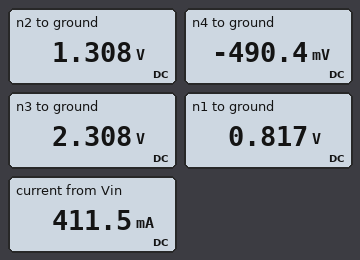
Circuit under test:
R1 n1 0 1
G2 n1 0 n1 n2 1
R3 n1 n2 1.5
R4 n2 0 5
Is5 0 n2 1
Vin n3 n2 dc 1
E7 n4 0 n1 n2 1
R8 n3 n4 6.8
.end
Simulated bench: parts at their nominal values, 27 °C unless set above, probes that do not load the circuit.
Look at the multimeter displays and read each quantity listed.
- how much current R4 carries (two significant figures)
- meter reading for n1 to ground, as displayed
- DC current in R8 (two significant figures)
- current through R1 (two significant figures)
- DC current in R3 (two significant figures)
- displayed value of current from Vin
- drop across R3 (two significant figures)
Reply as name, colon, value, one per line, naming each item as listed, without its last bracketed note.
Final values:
how much current R4 carries: 260 mA
meter reading for n1 to ground, as displayed: 0.817 V
DC current in R8: 410 mA
current through R1: 820 mA
DC current in R3: 330 mA
displayed value of current from Vin: 411.5 mA
drop across R3: 490 mV
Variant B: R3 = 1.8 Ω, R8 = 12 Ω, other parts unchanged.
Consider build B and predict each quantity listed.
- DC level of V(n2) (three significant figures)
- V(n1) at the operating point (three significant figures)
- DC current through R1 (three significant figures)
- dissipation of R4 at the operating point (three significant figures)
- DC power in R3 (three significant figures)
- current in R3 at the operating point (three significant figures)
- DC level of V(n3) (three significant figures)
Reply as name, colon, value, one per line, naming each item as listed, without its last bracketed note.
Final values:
DC level of V(n2): 1.72 V
V(n1) at the operating point: 1.05 V
DC current through R1: 1.05 A
dissipation of R4 at the operating point: 591 mW
DC power in R3: 251 mW
current in R3 at the operating point: 374 mA
DC level of V(n3): 2.72 V
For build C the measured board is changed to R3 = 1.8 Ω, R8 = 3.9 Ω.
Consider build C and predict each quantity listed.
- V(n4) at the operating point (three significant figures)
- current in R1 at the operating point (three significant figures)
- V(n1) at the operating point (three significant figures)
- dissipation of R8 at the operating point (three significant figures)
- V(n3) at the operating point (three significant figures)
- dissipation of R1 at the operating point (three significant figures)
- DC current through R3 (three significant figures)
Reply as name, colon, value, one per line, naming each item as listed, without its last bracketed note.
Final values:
V(n4) at the operating point: -376 mV
current in R1 at the operating point: 585 mA
V(n1) at the operating point: 585 mV
dissipation of R8 at the operating point: 1.40 W
V(n3) at the operating point: 1.96 V
dissipation of R1 at the operating point: 342 mW
DC current through R3: 209 mA
